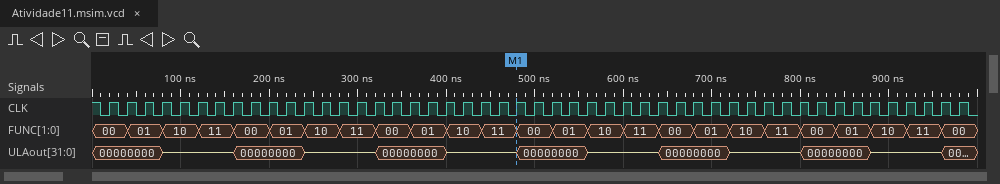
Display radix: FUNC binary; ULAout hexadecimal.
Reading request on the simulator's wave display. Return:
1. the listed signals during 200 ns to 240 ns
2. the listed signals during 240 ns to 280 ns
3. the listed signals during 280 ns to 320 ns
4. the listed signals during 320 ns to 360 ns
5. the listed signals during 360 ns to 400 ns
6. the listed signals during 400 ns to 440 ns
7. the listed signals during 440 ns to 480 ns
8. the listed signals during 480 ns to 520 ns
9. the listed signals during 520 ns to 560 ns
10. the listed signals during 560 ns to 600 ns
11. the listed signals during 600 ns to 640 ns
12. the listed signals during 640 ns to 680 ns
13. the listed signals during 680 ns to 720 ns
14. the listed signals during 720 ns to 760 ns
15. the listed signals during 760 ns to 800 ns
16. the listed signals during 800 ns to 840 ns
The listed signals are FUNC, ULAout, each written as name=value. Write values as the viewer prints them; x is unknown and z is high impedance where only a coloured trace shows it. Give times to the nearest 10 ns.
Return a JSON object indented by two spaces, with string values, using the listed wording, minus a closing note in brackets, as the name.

{
  "the listed signals during 200 ns to 240 ns": "FUNC=01, ULAout=00000000",
  "the listed signals during 240 ns to 280 ns": "FUNC=10, ULAout=z",
  "the listed signals during 280 ns to 320 ns": "FUNC=11, ULAout=z",
  "the listed signals during 320 ns to 360 ns": "FUNC=00, ULAout=00000000",
  "the listed signals during 360 ns to 400 ns": "FUNC=01, ULAout=00000000",
  "the listed signals during 400 ns to 440 ns": "FUNC=10, ULAout=z",
  "the listed signals during 440 ns to 480 ns": "FUNC=11, ULAout=z",
  "the listed signals during 480 ns to 520 ns": "FUNC=00, ULAout=00000000",
  "the listed signals during 520 ns to 560 ns": "FUNC=01, ULAout=00000000",
  "the listed signals during 560 ns to 600 ns": "FUNC=10, ULAout=z",
  "the listed signals during 600 ns to 640 ns": "FUNC=11, ULAout=z",
  "the listed signals during 640 ns to 680 ns": "FUNC=00, ULAout=00000000",
  "the listed signals during 680 ns to 720 ns": "FUNC=01, ULAout=00000000",
  "the listed signals during 720 ns to 760 ns": "FUNC=10, ULAout=z",
  "the listed signals during 760 ns to 800 ns": "FUNC=11, ULAout=z",
  "the listed signals during 800 ns to 840 ns": "FUNC=00, ULAout=00000000"
}
